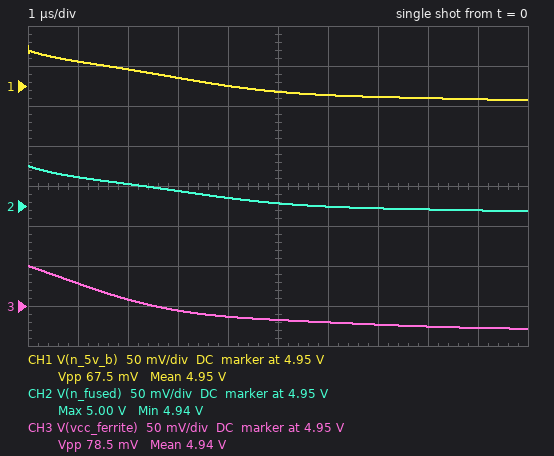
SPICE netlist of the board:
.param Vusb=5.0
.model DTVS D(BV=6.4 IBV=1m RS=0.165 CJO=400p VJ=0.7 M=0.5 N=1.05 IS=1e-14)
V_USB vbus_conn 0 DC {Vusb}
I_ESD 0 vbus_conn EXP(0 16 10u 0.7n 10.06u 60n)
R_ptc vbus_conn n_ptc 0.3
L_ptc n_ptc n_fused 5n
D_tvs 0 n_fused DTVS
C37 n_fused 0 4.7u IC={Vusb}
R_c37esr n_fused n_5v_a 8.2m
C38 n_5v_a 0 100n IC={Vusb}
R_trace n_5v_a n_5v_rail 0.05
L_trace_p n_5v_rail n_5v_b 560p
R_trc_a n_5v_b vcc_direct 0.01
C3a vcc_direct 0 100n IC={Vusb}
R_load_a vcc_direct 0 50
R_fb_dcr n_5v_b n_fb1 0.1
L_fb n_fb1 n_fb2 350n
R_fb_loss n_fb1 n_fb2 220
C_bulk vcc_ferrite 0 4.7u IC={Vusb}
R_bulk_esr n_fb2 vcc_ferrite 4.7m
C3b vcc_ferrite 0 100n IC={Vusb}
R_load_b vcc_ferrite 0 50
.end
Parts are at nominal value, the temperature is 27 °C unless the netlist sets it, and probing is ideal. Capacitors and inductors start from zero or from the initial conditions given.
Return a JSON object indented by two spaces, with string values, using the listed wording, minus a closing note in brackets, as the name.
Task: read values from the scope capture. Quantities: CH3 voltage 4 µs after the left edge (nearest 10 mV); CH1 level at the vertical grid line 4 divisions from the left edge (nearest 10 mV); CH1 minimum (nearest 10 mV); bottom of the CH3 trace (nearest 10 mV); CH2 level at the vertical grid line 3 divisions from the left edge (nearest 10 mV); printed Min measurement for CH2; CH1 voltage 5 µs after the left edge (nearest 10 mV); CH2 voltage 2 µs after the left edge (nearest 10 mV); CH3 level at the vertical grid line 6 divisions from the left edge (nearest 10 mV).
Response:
{
  "CH3 voltage 4 µs after the left edge": "4.94 V",
  "CH1 level at the vertical grid line 4 divisions from the left edge": "4.95 V",
  "CH1 minimum": "4.93 V",
  "bottom of the CH3 trace": "4.92 V",
  "CH2 level at the vertical grid line 3 divisions from the left edge": "4.97 V",
  "printed Min measurement for CH2": "4.94 V",
  "CH1 voltage 5 µs after the left edge": "4.94 V",
  "CH2 voltage 2 µs after the left edge": "4.98 V",
  "CH3 level at the vertical grid line 6 divisions from the left edge": "4.93 V"
}
